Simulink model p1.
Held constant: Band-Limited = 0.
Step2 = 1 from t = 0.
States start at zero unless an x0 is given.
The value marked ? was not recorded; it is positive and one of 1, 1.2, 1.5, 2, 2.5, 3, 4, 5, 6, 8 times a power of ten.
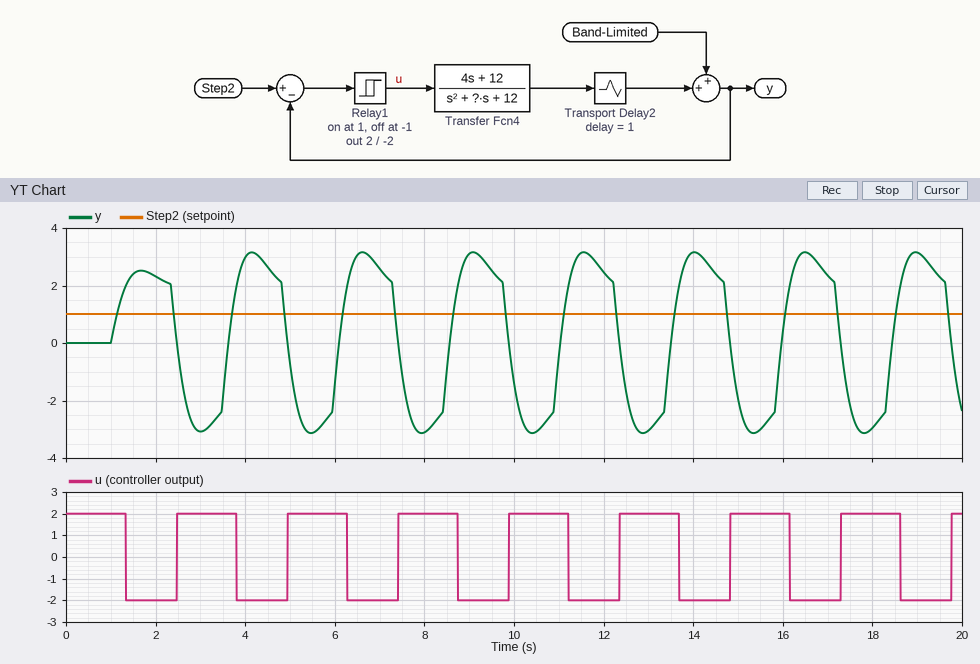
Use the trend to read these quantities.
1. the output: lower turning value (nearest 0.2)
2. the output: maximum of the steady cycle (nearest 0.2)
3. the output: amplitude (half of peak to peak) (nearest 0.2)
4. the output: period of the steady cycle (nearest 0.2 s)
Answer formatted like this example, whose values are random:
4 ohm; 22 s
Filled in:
-3.2; 3.2; 3.2; 2.4 s
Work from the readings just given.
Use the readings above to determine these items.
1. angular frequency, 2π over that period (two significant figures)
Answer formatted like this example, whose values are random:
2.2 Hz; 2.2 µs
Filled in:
2.6 rad/s
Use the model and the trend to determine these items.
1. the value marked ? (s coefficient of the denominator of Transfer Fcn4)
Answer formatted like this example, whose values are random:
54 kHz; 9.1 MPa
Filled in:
4
